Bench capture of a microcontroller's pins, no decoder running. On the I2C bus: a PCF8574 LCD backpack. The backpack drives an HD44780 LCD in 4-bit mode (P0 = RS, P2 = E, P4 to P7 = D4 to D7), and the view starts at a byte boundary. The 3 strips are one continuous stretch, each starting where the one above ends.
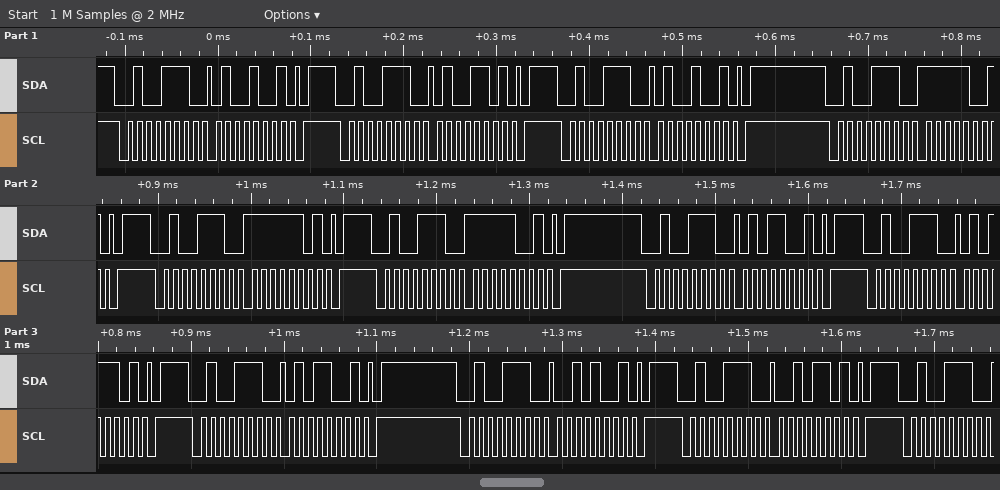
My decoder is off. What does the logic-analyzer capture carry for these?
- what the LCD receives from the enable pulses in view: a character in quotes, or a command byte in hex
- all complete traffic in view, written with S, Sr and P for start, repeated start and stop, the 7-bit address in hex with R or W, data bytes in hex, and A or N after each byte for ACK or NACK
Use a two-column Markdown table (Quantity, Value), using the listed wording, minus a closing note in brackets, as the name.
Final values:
| Quantity | Value |
|---|---|
| what the LCD receives from the enable pulses in view: a character in quotes, or a command byte in hex | 'O' |
| all complete traffic in view, written with S, Sr and P for start, repeated start and stop, the 7-bit address in hex with R or W, data bytes in hex, and A or N after each byte for ACK or NACK | S 27W A 49 A P S 27W A 4D A P S 27W A 49 A P S 27W A F9 A P S 27W A FD A P S 27W A F9 A P S 27W A 59 A P S 27W A 5D A P S 27W A 59 A P S 27W A 29 A P S 27W A 2D A P S 27W A |
